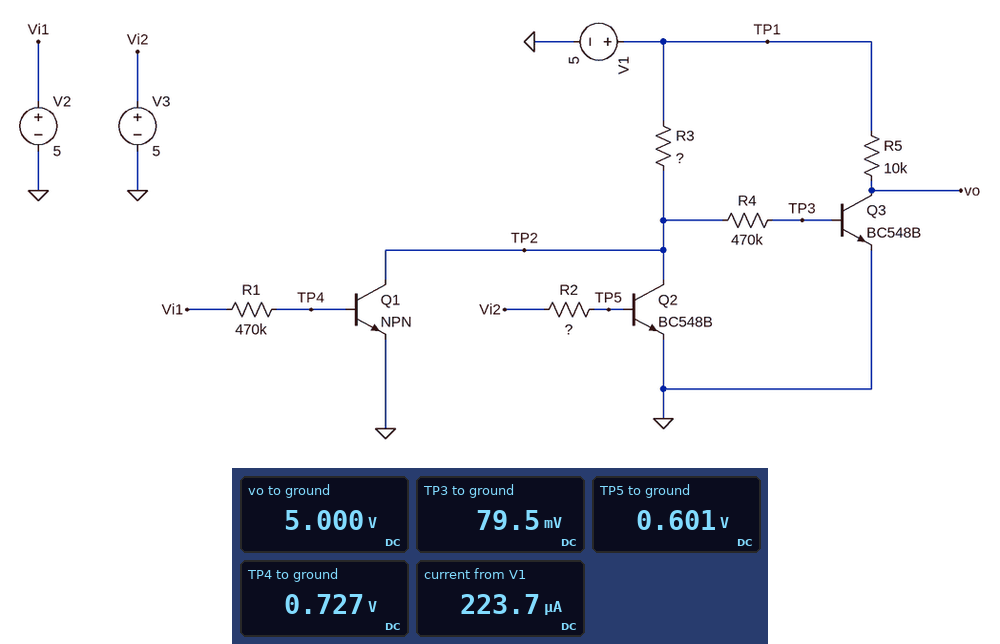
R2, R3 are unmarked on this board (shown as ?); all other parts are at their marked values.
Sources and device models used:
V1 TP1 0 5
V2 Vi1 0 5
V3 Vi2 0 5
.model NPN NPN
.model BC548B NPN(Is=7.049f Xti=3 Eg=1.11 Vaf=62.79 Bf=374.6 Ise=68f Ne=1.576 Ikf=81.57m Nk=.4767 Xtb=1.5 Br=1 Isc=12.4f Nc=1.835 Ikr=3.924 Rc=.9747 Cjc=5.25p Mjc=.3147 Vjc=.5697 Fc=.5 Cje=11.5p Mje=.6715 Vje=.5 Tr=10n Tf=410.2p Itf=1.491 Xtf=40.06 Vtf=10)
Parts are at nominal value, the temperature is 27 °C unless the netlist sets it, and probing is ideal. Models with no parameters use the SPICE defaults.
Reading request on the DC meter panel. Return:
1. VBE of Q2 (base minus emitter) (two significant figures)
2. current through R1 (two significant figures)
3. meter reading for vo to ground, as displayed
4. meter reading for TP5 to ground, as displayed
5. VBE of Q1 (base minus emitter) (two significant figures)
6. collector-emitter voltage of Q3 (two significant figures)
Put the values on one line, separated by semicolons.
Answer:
600 mV; 9.1 µA; 5.000 V; 0.601 V; 730 mV; 5.0 V
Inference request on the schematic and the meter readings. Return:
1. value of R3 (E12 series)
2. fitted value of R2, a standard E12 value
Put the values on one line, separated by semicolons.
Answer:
22 kΩ; 1 MΩ
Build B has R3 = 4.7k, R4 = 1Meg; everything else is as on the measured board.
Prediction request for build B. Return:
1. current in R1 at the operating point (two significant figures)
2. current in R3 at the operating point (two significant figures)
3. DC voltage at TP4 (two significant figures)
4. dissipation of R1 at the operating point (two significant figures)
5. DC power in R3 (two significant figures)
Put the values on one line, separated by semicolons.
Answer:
9.0 µA; 1.0 mA; 760 mV; 38 µW; 5.0 mW
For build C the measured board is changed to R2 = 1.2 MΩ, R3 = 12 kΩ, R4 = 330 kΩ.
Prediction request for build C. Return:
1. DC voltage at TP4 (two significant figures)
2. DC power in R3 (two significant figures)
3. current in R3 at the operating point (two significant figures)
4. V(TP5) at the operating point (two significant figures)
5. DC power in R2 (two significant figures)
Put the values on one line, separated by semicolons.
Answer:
740 mV; 2.0 mW; 410 µA; 610 mV; 16 µW
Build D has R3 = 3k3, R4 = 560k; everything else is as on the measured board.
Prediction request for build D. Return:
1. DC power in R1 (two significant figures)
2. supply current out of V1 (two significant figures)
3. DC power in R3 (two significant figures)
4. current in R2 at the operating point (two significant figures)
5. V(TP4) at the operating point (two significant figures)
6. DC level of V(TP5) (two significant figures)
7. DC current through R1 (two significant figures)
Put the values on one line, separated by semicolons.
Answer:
38 µW; 1.5 mA; 7.1 mW; 4.3 µA; 770 mV; 660 mV; 9.0 µA
